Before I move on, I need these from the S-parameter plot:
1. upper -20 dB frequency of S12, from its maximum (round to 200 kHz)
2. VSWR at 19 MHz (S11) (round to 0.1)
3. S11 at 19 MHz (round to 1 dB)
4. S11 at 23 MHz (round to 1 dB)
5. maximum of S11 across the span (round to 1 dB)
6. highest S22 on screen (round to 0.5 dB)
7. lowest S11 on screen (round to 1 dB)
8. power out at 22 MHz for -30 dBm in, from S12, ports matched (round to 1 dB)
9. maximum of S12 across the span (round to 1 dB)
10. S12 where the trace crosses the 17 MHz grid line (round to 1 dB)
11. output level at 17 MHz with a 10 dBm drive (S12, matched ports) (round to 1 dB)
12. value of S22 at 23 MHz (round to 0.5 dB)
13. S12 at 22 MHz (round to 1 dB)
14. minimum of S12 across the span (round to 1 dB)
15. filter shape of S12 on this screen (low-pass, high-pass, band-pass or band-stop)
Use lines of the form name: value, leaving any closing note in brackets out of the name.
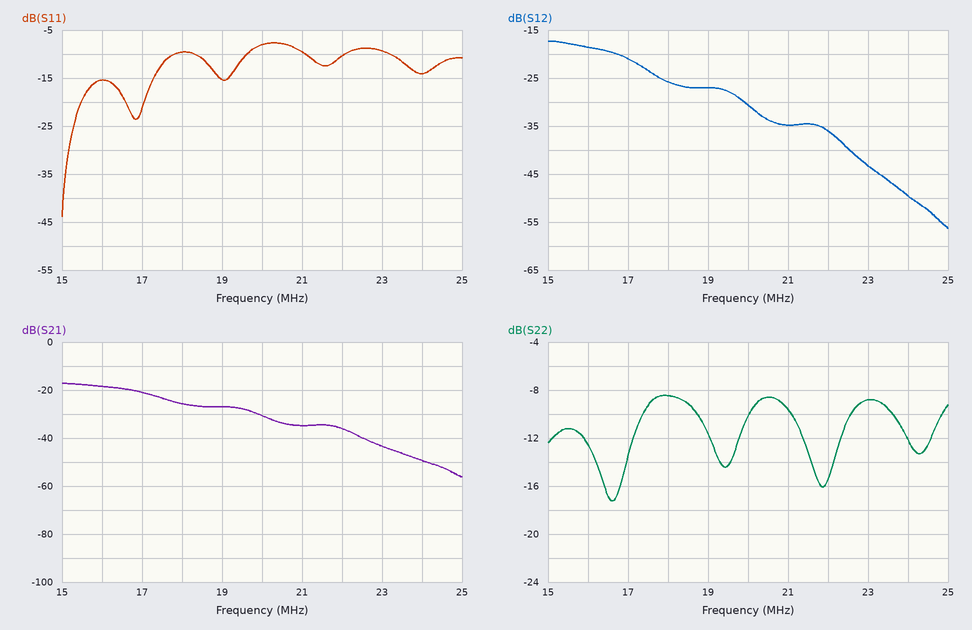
upper -20 dB frequency of S12, from its maximum: 22.2 MHz
VSWR at 19 MHz (S11): 1.4
S11 at 19 MHz: -15 dB
S11 at 23 MHz: -9 dB
maximum of S11 across the span: -8 dB
highest S22 on screen: -8.5 dB
lowest S11 on screen: -44 dB
power out at 22 MHz for -30 dBm in, from S12, ports matched: -66 dBm
maximum of S12 across the span: -17 dB
S12 where the trace crosses the 17 MHz grid line: -21 dB
output level at 17 MHz with a 10 dBm drive (S12, matched ports): -11 dBm
value of S22 at 23 MHz: -9.0 dB
S12 at 22 MHz: -36 dB
minimum of S12 across the span: -56 dB
filter shape of S12 on this screen: low-pass
